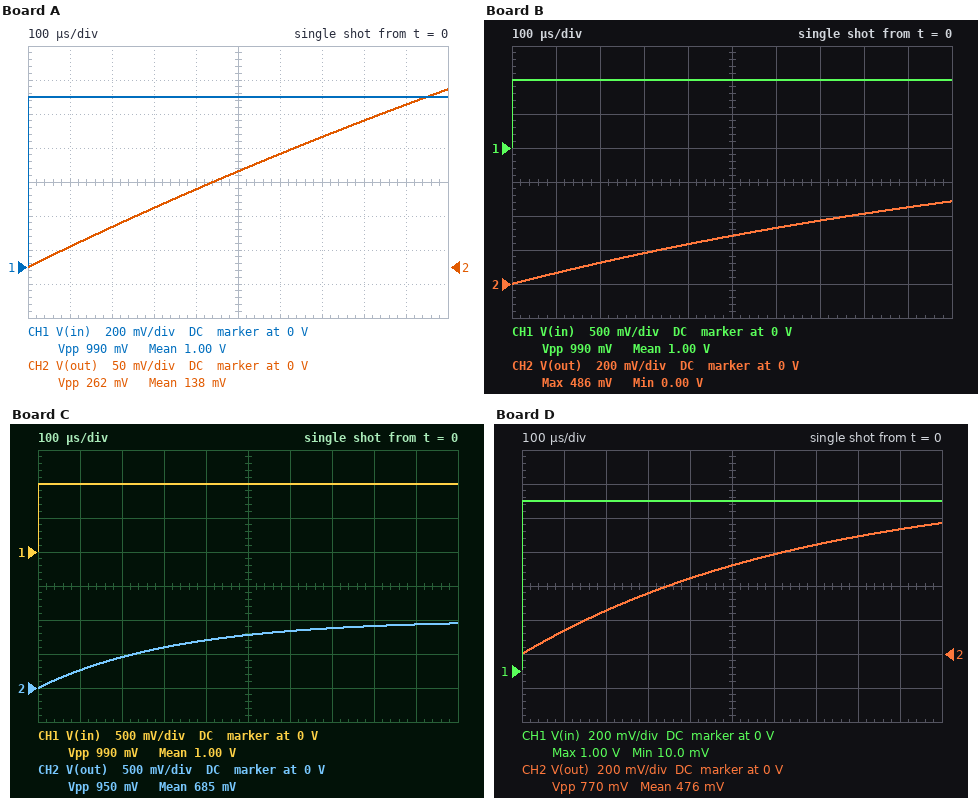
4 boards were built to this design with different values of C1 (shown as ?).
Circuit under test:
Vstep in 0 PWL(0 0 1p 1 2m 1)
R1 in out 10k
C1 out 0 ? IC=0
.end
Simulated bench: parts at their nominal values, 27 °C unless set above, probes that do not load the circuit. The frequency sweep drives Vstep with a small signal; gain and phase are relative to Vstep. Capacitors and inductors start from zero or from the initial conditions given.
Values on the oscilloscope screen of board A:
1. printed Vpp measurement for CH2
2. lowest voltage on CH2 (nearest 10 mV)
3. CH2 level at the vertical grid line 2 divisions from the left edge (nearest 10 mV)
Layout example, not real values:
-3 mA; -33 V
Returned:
262 mV; 0 V; 60 mV
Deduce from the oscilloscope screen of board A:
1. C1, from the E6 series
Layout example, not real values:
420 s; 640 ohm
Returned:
330 nF
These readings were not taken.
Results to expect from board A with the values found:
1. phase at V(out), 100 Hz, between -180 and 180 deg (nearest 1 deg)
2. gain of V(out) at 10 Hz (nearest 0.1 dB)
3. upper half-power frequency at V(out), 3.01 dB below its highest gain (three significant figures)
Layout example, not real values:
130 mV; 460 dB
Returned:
-64 deg; -0.2 dB; 48.2 Hz
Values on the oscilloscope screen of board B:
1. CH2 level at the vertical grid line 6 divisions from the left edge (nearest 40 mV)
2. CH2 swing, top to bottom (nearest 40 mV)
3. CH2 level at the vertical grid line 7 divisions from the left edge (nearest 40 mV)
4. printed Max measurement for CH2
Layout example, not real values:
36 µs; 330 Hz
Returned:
320 mV; 480 mV; 360 mV; 486 mV
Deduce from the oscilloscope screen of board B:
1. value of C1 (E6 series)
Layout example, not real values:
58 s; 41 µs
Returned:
150 nF
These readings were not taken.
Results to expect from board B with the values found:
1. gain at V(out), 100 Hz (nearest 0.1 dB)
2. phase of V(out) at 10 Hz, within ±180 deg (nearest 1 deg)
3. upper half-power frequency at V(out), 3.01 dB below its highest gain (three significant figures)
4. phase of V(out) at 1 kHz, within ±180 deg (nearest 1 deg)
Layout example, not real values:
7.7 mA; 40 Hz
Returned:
-2.8 dB; -5 deg; 106 Hz; -84 deg
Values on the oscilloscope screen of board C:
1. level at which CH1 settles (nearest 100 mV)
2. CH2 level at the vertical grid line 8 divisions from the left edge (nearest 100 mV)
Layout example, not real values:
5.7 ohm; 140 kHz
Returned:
1.0 V; 900 mV
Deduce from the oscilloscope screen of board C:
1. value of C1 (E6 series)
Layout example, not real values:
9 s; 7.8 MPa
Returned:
33 nF
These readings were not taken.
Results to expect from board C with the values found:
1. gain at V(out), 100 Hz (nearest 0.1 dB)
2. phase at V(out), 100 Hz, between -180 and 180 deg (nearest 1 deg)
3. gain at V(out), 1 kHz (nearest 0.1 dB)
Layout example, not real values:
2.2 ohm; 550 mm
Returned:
-0.2 dB; -12 deg; -7.2 dB
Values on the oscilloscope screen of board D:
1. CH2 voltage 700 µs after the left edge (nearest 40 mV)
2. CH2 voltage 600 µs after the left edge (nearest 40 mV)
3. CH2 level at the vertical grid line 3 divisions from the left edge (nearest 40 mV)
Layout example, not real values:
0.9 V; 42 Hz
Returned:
640 mV; 600 mV; 360 mV
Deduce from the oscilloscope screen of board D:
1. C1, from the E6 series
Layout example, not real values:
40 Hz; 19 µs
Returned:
68 nF
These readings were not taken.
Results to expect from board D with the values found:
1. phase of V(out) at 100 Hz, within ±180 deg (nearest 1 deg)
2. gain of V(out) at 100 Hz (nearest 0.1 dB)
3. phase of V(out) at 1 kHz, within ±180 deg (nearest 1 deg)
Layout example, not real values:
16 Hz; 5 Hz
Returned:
-23 deg; -0.7 dB; -77 deg
